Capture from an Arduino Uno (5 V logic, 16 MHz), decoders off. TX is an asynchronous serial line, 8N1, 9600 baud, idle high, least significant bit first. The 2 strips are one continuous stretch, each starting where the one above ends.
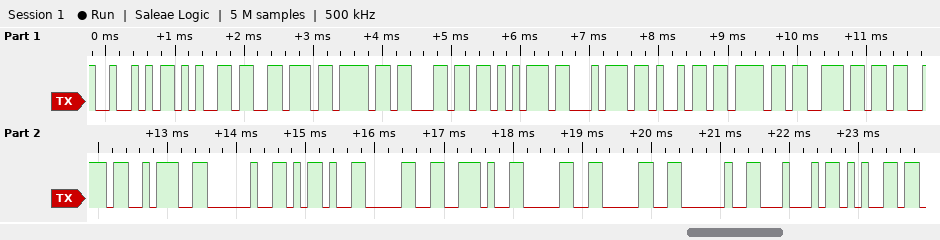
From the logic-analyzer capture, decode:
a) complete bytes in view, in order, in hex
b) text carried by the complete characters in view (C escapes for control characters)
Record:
52 65 76 6F 6C 75 74 69 6F 6E 73 3A 20 2D 30 2E 30 30 20 44 65
"Revolutions: -0.00 De"
